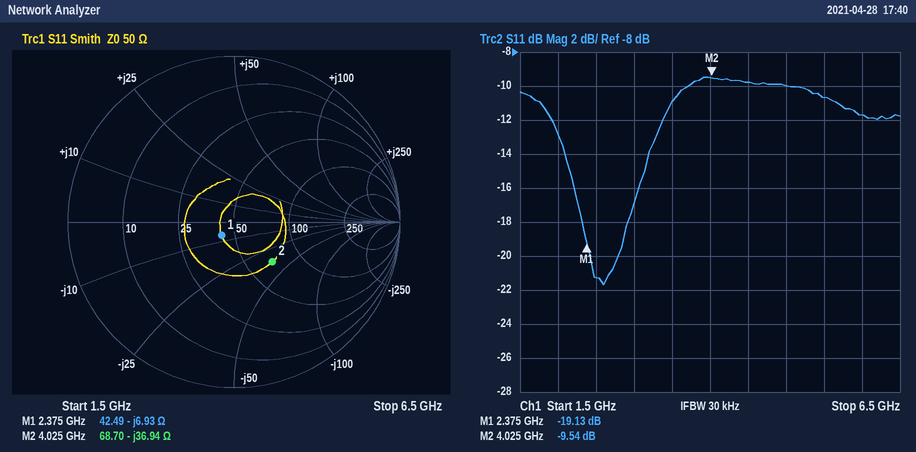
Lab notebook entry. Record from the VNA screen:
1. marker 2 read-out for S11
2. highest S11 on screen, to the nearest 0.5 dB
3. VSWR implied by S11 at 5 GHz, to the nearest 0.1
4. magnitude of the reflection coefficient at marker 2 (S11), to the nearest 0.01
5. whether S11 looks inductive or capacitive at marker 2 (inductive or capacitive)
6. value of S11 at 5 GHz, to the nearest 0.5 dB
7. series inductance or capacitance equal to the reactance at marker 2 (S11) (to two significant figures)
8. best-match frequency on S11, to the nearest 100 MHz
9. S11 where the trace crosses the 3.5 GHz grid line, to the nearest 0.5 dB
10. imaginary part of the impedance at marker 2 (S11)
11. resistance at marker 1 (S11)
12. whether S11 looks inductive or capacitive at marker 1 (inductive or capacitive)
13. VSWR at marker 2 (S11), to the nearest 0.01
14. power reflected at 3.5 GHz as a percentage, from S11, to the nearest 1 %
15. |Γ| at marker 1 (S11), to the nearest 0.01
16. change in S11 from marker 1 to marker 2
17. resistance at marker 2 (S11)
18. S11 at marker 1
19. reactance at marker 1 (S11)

-9.54 dB
-9.5 dB
1.9
0.33
capacitive
-10.0 dB
1.1 pF
2.6 GHz
-11.0 dB
-36.94 Ω
42.49 Ω
capacitive
2.00
8 %
0.11
9.59 dB
68.70 Ω
-19.13 dB
-6.93 Ω
